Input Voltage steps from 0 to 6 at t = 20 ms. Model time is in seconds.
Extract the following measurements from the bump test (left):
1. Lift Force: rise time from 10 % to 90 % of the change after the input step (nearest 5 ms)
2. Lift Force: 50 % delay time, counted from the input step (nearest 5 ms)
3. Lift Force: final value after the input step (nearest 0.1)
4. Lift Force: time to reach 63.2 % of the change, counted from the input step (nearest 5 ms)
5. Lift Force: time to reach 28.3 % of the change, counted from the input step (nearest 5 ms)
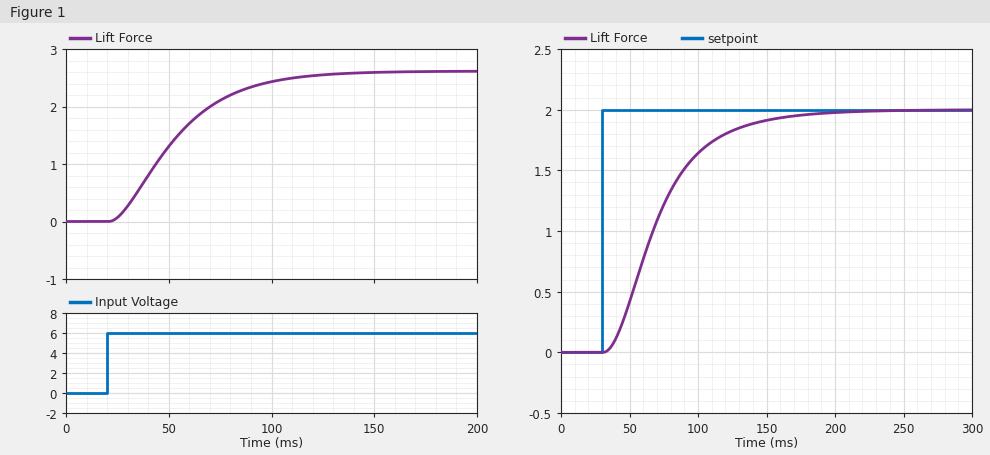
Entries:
60 ms
30 ms
2.6
40 ms
20 ms
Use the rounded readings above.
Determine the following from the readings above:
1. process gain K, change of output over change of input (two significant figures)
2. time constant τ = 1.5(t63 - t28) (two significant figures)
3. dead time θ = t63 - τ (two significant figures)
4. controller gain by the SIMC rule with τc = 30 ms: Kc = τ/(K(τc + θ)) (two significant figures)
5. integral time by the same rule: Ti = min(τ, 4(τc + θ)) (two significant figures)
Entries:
0.43
30 ms
10 ms
1.7
30 ms
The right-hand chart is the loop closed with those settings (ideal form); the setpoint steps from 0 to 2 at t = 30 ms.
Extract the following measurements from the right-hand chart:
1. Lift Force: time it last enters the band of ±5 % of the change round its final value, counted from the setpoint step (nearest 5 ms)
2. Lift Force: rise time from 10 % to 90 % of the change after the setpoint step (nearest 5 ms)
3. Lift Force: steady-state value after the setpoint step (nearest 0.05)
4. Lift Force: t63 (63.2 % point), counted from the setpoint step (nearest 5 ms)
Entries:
115 ms
75 ms
2.00
45 ms
